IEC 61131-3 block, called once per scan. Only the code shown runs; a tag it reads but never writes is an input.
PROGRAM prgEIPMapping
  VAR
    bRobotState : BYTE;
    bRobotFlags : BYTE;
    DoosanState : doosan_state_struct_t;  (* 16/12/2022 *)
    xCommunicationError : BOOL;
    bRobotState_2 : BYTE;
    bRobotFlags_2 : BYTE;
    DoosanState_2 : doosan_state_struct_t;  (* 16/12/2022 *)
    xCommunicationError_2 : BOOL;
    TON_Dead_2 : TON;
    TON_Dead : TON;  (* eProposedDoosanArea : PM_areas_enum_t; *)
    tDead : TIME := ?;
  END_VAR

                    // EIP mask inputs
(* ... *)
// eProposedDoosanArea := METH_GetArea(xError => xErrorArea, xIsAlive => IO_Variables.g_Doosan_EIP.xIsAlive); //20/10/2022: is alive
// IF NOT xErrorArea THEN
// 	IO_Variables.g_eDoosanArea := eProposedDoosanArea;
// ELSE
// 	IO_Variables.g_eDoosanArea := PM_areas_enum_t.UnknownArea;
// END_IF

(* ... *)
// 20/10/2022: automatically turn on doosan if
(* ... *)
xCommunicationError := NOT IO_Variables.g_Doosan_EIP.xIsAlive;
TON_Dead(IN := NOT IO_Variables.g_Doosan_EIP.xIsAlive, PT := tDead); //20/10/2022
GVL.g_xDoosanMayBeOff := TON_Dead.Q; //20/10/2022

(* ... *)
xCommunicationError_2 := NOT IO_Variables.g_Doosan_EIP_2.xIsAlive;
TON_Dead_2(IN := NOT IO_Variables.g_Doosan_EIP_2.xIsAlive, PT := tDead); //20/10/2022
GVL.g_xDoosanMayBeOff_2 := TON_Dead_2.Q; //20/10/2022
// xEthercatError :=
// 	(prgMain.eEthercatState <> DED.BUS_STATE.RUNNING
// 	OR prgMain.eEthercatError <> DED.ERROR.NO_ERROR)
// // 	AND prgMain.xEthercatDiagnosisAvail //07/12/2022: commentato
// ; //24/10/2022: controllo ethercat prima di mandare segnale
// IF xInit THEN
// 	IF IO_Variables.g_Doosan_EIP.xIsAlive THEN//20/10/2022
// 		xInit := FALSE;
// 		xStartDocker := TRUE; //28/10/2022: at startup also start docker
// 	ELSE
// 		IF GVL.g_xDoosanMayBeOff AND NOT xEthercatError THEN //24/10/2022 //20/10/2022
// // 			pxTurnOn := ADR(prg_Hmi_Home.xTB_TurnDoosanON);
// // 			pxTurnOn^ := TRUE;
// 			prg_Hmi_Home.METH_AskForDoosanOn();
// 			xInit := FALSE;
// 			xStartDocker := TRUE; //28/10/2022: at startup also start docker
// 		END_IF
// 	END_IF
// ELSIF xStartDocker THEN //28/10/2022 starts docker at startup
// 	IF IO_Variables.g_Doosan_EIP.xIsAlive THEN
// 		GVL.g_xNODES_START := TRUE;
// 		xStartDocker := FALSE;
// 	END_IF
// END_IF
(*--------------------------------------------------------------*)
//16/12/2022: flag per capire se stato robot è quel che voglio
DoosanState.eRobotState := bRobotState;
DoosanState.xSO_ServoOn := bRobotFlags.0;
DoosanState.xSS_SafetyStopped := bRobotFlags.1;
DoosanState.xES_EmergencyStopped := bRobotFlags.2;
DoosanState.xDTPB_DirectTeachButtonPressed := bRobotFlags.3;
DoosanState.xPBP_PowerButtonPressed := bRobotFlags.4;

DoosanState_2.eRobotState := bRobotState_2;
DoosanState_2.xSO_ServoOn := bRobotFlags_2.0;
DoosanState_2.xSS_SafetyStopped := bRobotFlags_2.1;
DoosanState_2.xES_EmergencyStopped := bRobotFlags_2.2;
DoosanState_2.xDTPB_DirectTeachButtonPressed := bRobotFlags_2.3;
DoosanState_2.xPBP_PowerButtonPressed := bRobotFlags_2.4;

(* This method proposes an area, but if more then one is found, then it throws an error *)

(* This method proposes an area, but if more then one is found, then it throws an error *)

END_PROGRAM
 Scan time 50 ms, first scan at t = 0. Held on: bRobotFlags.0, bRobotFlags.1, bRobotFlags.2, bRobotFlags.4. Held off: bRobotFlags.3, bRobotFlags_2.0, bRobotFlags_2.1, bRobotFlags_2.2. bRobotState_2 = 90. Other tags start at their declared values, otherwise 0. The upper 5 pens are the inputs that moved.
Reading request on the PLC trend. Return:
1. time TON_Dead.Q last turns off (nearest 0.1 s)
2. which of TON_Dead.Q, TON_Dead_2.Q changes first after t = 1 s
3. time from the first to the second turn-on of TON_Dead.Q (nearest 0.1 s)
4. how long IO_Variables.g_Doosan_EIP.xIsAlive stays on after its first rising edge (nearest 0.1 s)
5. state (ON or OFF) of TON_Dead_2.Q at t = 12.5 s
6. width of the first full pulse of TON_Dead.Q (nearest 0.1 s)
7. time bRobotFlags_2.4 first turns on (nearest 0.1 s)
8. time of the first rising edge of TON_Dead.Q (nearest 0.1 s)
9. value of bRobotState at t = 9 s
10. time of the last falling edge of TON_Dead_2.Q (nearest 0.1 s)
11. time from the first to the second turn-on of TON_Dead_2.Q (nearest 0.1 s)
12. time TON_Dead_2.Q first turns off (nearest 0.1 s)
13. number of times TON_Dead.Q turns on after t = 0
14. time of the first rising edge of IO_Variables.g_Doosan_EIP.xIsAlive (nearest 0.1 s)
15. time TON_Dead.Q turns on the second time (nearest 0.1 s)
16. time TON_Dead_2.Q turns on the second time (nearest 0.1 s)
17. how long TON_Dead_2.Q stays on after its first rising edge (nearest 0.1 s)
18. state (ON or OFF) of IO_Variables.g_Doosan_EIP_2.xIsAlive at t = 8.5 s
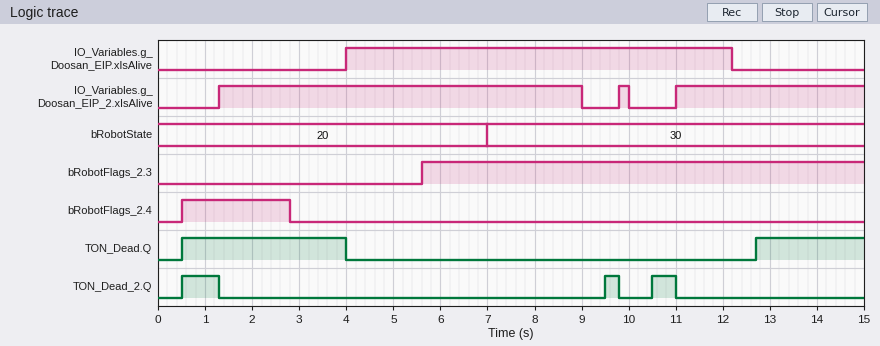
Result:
4.0 s
TON_Dead_2.Q
12.2 s
8.2 s
OFF
3.5 s
0.5 s
0.5 s
30
11.0 s
9.0 s
1.3 s
2
4.0 s
12.7 s
9.5 s
0.8 s
ON
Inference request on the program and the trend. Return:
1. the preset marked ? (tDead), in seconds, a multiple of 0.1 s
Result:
0.5 s
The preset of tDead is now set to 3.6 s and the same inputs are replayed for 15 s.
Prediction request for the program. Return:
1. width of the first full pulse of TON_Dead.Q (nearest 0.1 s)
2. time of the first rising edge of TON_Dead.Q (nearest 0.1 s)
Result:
0.4 s
3.6 s
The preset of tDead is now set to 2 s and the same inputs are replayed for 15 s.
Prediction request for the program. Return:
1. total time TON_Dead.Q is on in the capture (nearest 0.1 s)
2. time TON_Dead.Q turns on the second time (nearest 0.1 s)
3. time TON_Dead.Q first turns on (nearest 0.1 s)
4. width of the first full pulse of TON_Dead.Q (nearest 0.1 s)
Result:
2.8 s
14.2 s
2.0 s
2.0 s
